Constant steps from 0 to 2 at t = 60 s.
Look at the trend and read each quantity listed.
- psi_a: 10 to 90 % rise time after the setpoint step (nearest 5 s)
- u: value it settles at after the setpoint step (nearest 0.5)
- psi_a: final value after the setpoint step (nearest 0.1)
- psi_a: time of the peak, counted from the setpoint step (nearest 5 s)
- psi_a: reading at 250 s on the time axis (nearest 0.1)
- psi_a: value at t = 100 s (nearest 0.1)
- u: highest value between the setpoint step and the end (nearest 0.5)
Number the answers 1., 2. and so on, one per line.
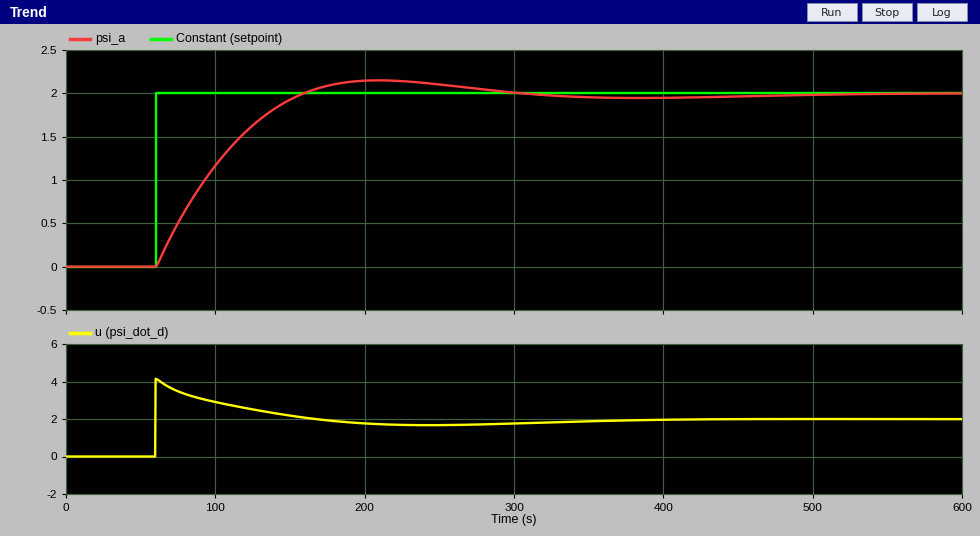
1. 70 s
2. 2.0
3. 2.0
4. 150 s
5. 2.1
6. 1.2
7. 4.0
